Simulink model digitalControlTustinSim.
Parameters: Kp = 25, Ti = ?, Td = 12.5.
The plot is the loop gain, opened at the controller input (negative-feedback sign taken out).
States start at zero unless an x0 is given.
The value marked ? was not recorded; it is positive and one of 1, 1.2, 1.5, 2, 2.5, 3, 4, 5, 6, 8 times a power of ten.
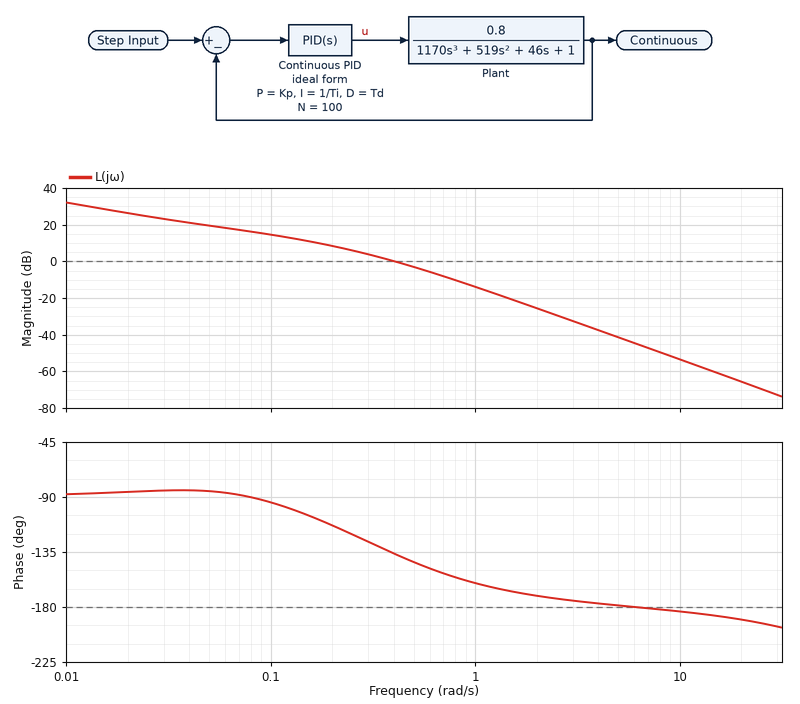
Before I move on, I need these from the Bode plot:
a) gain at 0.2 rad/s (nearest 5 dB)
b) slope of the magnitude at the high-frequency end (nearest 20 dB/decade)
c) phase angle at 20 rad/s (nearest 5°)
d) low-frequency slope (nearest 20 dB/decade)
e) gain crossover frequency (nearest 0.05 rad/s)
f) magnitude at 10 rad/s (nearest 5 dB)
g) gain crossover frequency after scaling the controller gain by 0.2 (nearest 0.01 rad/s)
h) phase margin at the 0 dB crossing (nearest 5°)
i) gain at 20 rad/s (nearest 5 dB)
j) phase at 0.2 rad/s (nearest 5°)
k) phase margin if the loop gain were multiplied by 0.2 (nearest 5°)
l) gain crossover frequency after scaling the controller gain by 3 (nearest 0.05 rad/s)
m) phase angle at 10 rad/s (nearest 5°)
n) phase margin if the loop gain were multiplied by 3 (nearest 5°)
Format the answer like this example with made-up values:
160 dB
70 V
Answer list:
10 dB
-40 dB/decade
-190°
-20 dB/decade
0.40 rad/s
-55 dB
0.11 rad/s
45°
-65 dB
-115°
85°
0.75 rad/s
-185°
25°
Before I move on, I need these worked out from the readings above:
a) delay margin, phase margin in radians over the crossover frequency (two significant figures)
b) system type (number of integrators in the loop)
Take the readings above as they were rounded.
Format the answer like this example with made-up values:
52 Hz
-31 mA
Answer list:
2.0 s
1
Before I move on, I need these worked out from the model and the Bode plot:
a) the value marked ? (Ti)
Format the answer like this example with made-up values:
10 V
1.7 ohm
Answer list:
50
